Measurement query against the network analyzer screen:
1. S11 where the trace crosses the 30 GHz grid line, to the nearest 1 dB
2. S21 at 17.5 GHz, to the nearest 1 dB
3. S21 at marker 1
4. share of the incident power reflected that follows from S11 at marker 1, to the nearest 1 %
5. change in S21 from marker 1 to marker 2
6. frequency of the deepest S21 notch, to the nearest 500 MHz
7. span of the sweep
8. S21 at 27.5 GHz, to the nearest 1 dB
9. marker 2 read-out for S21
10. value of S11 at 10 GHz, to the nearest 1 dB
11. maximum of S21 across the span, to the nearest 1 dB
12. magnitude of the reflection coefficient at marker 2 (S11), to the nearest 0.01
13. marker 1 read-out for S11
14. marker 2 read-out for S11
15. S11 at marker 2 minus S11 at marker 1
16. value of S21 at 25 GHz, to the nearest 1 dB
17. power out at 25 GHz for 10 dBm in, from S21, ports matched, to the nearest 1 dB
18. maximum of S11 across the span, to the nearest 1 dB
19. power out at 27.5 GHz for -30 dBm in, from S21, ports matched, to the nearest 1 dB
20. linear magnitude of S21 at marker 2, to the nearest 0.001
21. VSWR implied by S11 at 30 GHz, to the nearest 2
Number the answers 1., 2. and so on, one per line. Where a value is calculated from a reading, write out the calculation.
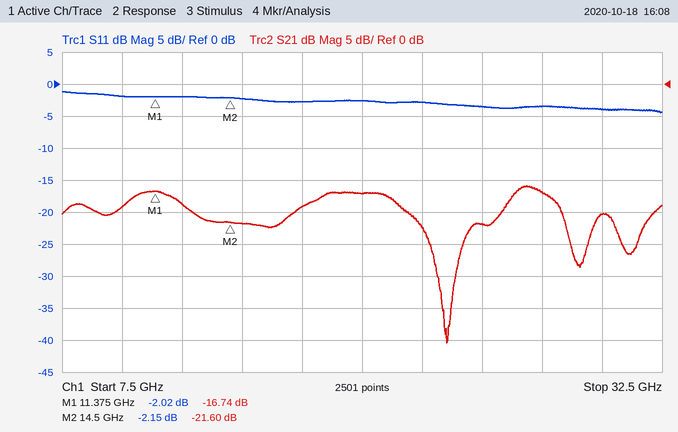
1. -4 dB
2. -19 dB
3. -16.74 dB
4. 10^(-2.02/10) ≈ 63 %
5. -21.6 − (-16.74) = -4.86 dB
6. 23.5 GHz
7. 25 GHz
8. -17 dB
9. -21.60 dB
10. -2 dB
11. -16 dB
12. 10^(-2.15/20) ≈ 0.78
13. -2.02 dB
14. -2.15 dB
15. -2.15 − (-2.02) = -0.13 dB
16. -22 dB
17. 10 dBm + (-22 dB) = -12 dBm
18. -1 dB
19. -30 dBm + (-17 dB) = -47 dBm
20. 10^(-21.6/20) ≈ 0.083
21. |Γ| = 10^(-4/20) = 0.6310; VSWR = (1 + 0.6310)/(1 − 0.6310) ≈ 4
